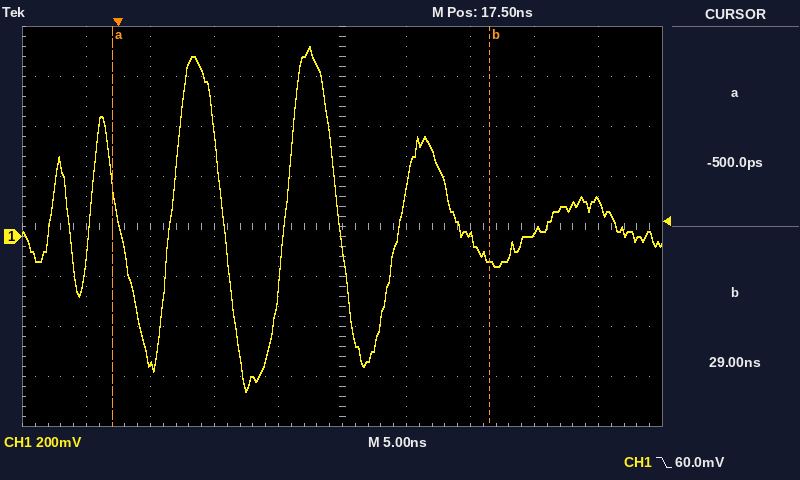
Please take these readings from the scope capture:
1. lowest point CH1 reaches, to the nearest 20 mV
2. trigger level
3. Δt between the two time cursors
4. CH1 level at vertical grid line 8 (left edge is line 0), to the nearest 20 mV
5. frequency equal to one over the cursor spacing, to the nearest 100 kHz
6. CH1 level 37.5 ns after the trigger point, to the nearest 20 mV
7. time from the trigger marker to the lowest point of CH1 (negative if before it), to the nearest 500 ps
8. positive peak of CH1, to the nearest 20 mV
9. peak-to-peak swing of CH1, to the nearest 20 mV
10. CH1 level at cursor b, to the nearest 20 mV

-620 mV
60.0 mV
29.5 ns
20 mV
33.9 MHz
140 mV
+10.0 ns
760 mV
1.38 V
-100 mV
